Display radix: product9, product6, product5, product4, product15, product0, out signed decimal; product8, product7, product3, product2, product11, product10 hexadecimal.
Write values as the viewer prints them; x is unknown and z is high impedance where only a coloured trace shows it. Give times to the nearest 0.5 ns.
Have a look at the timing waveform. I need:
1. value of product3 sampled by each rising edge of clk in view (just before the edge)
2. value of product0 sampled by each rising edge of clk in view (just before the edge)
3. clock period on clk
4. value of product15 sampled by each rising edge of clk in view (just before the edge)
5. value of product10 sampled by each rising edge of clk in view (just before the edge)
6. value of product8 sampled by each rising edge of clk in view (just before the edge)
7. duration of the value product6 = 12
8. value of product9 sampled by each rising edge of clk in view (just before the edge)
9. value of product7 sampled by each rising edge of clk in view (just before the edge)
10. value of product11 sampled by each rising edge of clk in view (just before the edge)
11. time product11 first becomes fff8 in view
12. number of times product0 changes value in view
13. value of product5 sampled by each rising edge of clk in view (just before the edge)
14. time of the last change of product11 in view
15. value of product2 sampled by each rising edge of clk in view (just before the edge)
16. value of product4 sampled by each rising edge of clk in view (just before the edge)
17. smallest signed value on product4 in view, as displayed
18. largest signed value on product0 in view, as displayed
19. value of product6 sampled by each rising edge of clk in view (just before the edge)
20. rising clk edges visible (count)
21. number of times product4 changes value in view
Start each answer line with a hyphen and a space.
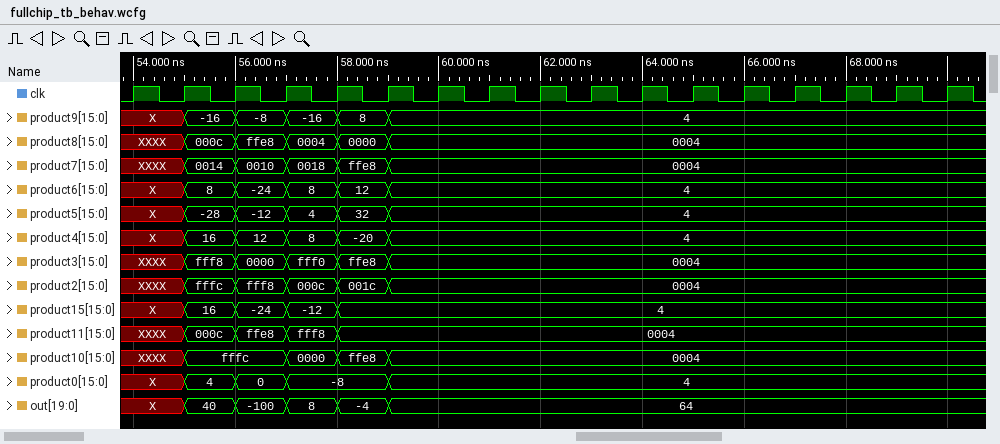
- XXXX, XXXX, fff8, 0000, fff0, ffe8, 0004, 0004, 0004, 0004, 0004, 0004, 0004, 0004, 0004, 0004, 0004
- X, X, 4, 0, -8, -8, 4, 4, 4, 4, 4, 4, 4, 4, 4, 4, 4
- 1 ns
- X, X, 16, -24, -12, 4, 4, 4, 4, 4, 4, 4, 4, 4, 4, 4, 4
- XXXX, XXXX, fffc, fffc, 0000, ffe8, 0004, 0004, 0004, 0004, 0004, 0004, 0004, 0004, 0004, 0004, 0004
- XXXX, XXXX, 000c, ffe8, 0004, 0000, 0004, 0004, 0004, 0004, 0004, 0004, 0004, 0004, 0004, 0004, 0004
- 1 ns
- X, X, -16, -8, -16, 8, 4, 4, 4, 4, 4, 4, 4, 4, 4, 4, 4
- XXXX, XXXX, 0014, 0010, 0018, ffe8, 0004, 0004, 0004, 0004, 0004, 0004, 0004, 0004, 0004, 0004, 0004
- XXXX, XXXX, 000c, ffe8, fff8, 0004, 0004, 0004, 0004, 0004, 0004, 0004, 0004, 0004, 0004, 0004, 0004
- 57 ns
- 4
- X, X, -28, -12, 4, 32, 4, 4, 4, 4, 4, 4, 4, 4, 4, 4, 4
- 58 ns
- XXXX, XXXX, fffc, fff8, 000c, 001c, 0004, 0004, 0004, 0004, 0004, 0004, 0004, 0004, 0004, 0004, 0004
- X, X, 16, 12, 8, -20, 4, 4, 4, 4, 4, 4, 4, 4, 4, 4, 4
- -20
- 4
- X, X, 8, -24, 8, 12, 4, 4, 4, 4, 4, 4, 4, 4, 4, 4, 4
- 17
- 5
